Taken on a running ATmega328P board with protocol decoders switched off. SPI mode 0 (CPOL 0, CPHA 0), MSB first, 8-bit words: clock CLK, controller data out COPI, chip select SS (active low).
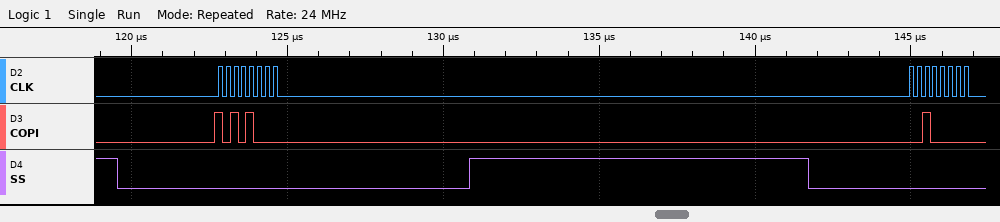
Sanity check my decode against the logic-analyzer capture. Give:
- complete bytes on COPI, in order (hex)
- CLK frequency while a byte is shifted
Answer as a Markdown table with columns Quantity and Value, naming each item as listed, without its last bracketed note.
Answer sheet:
| Quantity | Value |
|---|---|
| complete bytes on COPI, in order | A8 20 |
| CLK frequency while a byte is shifted | 4 MHz |
